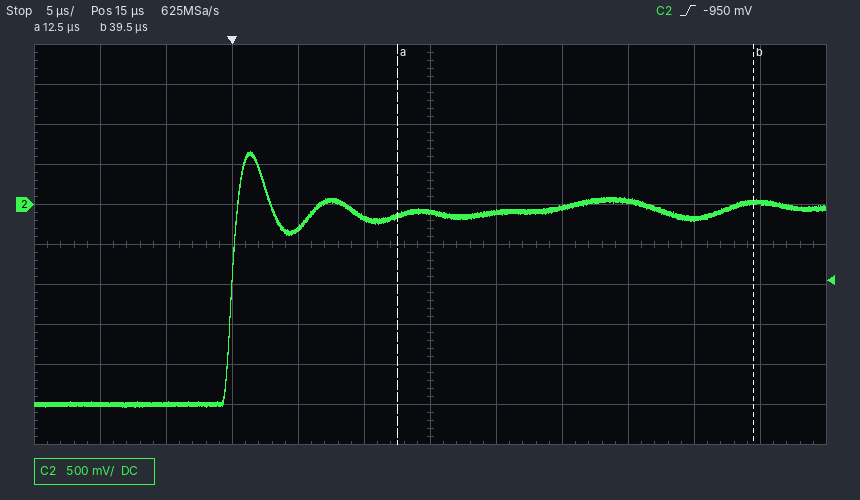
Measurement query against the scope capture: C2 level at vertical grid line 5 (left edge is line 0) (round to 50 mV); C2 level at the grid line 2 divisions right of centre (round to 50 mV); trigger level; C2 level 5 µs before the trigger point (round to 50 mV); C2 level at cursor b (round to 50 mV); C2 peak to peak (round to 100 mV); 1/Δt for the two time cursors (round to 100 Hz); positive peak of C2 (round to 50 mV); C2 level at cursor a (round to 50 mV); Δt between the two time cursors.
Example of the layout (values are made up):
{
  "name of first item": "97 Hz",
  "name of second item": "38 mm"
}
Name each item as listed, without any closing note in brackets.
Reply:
{
  "C2 level at vertical grid line 5 (left edge is line 0)": "-150 mV",
  "C2 level at the grid line 2 divisions right of centre": "-50 mV",
  "trigger level": "-950 mV",
  "C2 level 5 µs before the trigger point": "-2.50 V",
  "C2 level at cursor b": "50 mV",
  "C2 peak to peak": "3.20 V",
  "1/Δt for the two time cursors": "37.0 kHz",
  "positive peak of C2": "650 mV",
  "C2 level at cursor a": "-150 mV",
  "Δt between the two time cursors": "27.0 µs"
}
